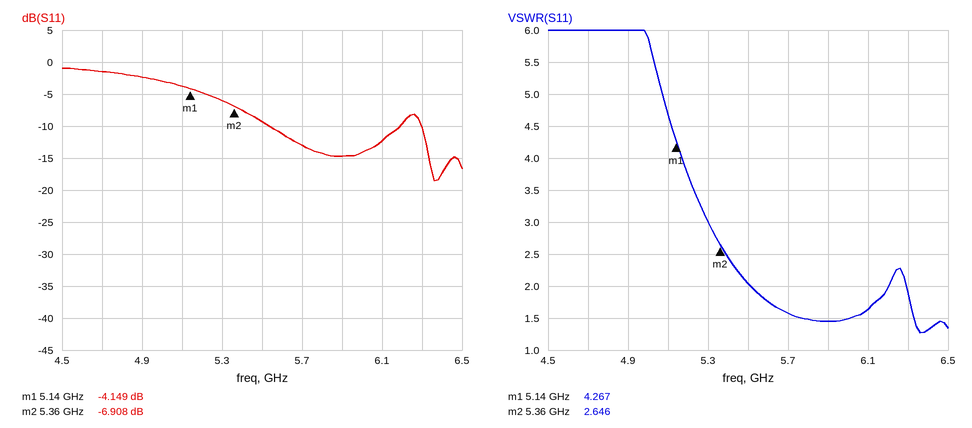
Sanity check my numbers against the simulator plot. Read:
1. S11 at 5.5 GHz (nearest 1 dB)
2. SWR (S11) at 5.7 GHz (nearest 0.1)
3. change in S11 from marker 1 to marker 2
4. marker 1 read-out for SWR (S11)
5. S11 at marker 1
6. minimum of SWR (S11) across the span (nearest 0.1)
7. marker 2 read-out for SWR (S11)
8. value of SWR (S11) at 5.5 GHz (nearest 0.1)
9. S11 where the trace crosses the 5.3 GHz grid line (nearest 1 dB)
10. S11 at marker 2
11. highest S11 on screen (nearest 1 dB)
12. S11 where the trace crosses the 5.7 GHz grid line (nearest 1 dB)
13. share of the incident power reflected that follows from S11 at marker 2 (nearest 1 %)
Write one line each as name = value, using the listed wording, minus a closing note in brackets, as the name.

S11 at 5.5 GHz = -9 dB
SWR (S11) at 5.7 GHz = 1.6
change in S11 from marker 1 to marker 2 = -2.759 dB
marker 1 read-out for SWR = 4.267
S11 at marker 1 = -4.149 dB
minimum of SWR (S11) across the span = 1.3
marker 2 read-out for SWR = 2.646
value of SWR (S11) at 5.5 GHz = 2.0
S11 where the trace crosses the 5.3 GHz grid line = -6 dB
S11 at marker 2 = -6.908 dB
highest S11 on screen = -1 dB
S11 where the trace crosses the 5.7 GHz grid line = -13 dB
share of the incident power reflected that follows from S11 at marker 2 = 20 %
